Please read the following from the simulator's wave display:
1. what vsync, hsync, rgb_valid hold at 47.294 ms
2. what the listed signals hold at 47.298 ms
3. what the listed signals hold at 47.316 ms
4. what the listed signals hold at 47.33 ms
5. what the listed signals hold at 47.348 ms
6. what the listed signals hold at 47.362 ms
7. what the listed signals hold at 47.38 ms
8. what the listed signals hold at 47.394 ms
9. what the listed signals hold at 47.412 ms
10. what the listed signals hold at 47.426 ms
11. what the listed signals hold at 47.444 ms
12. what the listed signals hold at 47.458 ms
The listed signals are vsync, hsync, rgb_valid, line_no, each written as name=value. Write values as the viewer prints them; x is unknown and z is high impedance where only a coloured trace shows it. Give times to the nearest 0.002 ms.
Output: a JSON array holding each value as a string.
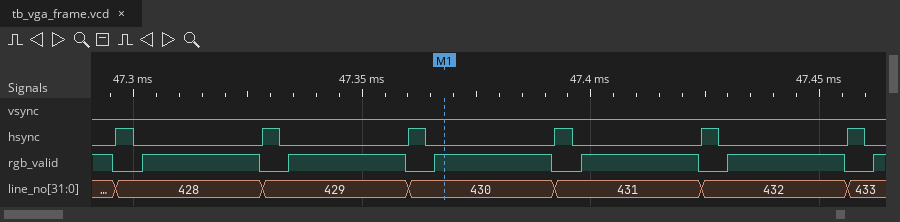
["vsync=0, hsync=0, rgb_valid=1", "vsync=0, hsync=1, rgb_valid=0, line_no=428", "vsync=0, hsync=0, rgb_valid=1, line_no=428", "vsync=0, hsync=1, rgb_valid=0, line_no=429", "vsync=0, hsync=0, rgb_valid=1, line_no=429", "vsync=0, hsync=1, rgb_valid=0, line_no=430", "vsync=0, hsync=0, rgb_valid=1, line_no=430", "vsync=0, hsync=1, rgb_valid=0, line_no=431", "vsync=0, hsync=0, rgb_valid=1, line_no=431", "vsync=0, hsync=1, rgb_valid=0, line_no=432", "vsync=0, hsync=0, rgb_valid=1, line_no=432", "vsync=0, hsync=1, rgb_valid=0, line_no=433"]
